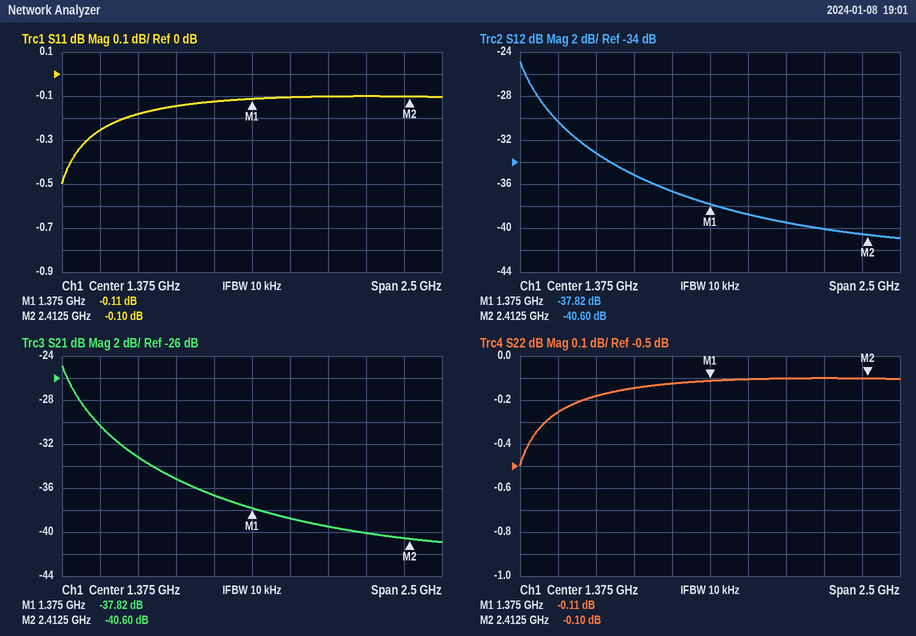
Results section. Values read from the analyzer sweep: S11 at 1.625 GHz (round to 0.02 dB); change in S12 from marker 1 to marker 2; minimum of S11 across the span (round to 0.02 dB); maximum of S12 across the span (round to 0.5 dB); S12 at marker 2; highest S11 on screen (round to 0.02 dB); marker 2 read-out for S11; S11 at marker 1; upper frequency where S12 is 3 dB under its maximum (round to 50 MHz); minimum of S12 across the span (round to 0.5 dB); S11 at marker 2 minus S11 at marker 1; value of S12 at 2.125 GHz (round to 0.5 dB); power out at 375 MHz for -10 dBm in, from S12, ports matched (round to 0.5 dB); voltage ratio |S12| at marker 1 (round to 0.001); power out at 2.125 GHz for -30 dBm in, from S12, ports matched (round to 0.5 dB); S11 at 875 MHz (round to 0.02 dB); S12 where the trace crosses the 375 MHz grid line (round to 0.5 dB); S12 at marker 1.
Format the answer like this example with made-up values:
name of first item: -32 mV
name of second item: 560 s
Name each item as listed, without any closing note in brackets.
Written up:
S11 at 1.625 GHz: -0.10 dB
change in S12 from marker 1 to marker 2: -2.78 dB
minimum of S11 across the span: -0.50 dB
maximum of S12 across the span: -25.0 dB
S12 at marker 2: -40.60 dB
highest S11 on screen: -0.10 dB
marker 2 read-out for S11: -0.10 dB
S11 at marker 1: -0.11 dB
upper frequency where S12 is 3 dB under its maximum: 250 MHz
minimum of S12 across the span: -41.0 dB
S11 at marker 2 minus S11 at marker 1: 0.01 dB
value of S12 at 2.125 GHz: -40.0 dB
power out at 375 MHz for -10 dBm in, from S12, ports matched: -40.5 dBm
voltage ratio |S12| at marker 1: 0.013
power out at 2.125 GHz for -30 dBm in, from S12, ports matched: -70.0 dBm
S11 at 875 MHz: -0.14 dB
S12 where the trace crosses the 375 MHz grid line: -30.5 dB
S12 at marker 1: -37.82 dB
